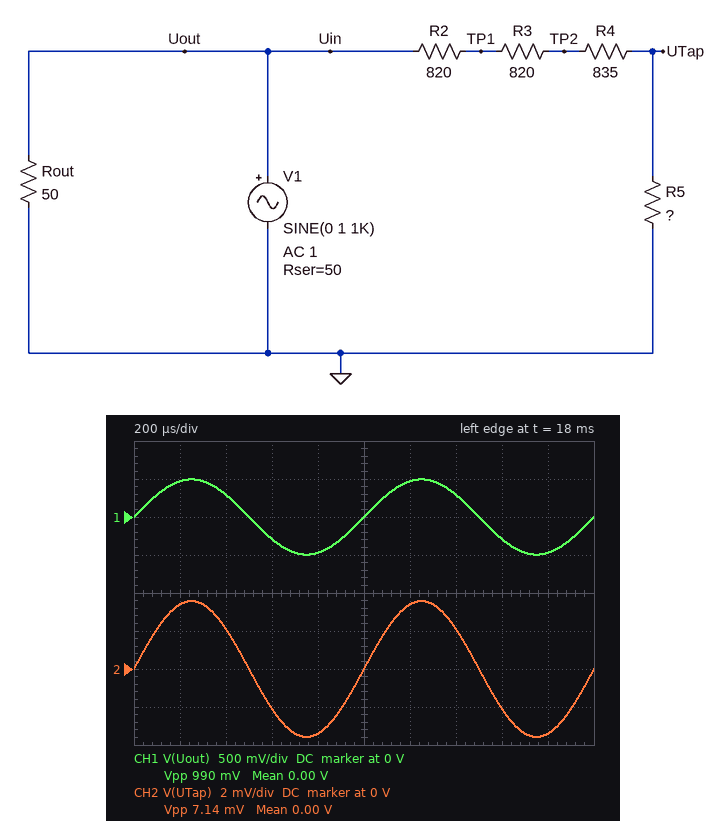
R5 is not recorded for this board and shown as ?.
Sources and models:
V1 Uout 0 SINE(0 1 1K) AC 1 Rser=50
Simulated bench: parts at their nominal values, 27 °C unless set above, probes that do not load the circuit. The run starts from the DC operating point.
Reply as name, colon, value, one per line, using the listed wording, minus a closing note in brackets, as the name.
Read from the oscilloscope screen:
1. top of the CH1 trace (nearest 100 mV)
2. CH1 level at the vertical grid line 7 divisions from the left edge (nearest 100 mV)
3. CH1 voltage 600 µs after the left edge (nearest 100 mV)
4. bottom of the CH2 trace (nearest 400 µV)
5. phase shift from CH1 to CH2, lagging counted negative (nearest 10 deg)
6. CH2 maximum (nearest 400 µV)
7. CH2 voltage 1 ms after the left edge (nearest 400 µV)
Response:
top of the CH1 trace: 500 mV
CH1 level at the vertical grid line 7 divisions from the left edge: 300 mV
CH1 voltage 600 µs after the left edge: -300 mV
bottom of the CH2 trace: -3.6 mV
phase shift from CH1 to CH2, lagging counted negative: 0 deg
CH2 maximum: 3.6 mV
CH2 voltage 1 ms after the left edge: 0 V
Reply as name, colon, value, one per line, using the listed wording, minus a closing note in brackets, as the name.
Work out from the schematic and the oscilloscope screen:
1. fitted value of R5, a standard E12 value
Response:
fitted value of R5, a standard E12 value: 18 Ω
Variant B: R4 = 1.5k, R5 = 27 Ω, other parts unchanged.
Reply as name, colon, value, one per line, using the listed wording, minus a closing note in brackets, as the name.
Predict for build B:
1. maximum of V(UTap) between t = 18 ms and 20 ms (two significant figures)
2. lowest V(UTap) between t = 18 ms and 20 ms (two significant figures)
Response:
maximum of V(UTap) between t = 18 ms and 20 ms: 4.2 mV
lowest V(UTap) between t = 18 ms and 20 ms: -4.2 mV
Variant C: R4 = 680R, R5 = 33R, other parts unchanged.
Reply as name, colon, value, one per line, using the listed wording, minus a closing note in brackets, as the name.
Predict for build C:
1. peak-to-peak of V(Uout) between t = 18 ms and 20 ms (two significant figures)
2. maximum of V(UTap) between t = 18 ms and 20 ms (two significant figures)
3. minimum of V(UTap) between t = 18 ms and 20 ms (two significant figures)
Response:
peak-to-peak of V(Uout) between t = 18 ms and 20 ms: 990 mV
maximum of V(UTap) between t = 18 ms and 20 ms: 6.9 mV
minimum of V(UTap) between t = 18 ms and 20 ms: -6.9 mV
